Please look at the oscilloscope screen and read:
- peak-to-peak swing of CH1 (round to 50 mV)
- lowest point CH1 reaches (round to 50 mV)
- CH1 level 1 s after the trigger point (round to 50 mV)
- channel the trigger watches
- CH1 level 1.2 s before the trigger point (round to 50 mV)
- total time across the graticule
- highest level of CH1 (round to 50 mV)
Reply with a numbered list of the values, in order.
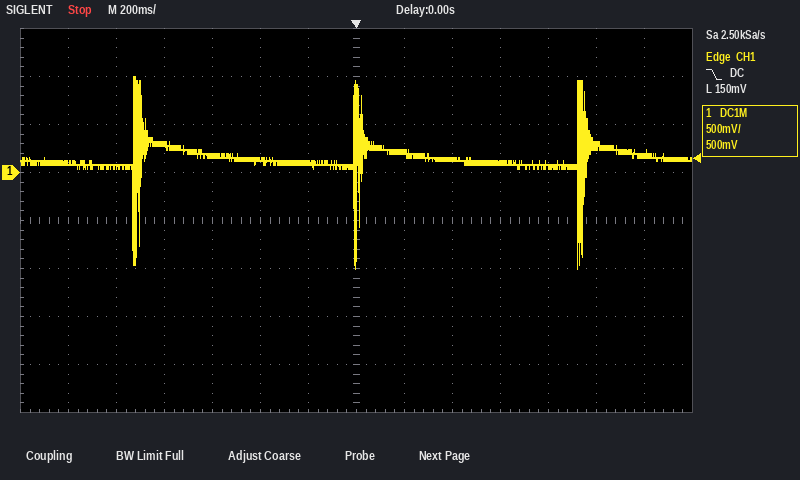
1. 2.00 V
2. -1.00 V
3. 300 mV
4. CH1
5. 100 mV
6. 2.8 s
7. 1.00 V
